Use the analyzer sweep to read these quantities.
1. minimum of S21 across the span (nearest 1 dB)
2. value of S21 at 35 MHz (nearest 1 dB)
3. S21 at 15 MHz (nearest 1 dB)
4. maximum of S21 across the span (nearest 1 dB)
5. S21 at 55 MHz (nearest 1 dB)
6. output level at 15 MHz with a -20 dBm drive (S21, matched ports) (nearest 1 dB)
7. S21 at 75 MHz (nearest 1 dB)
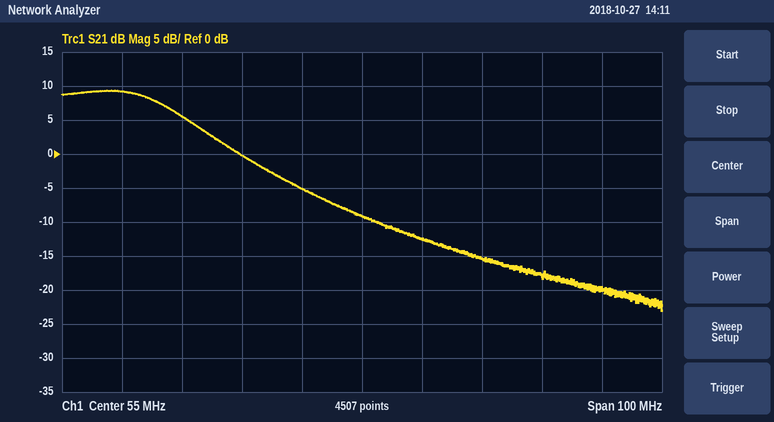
-23 dB
0 dB
9 dB
9 dB
-9 dB
-11 dBm
-15 dB
